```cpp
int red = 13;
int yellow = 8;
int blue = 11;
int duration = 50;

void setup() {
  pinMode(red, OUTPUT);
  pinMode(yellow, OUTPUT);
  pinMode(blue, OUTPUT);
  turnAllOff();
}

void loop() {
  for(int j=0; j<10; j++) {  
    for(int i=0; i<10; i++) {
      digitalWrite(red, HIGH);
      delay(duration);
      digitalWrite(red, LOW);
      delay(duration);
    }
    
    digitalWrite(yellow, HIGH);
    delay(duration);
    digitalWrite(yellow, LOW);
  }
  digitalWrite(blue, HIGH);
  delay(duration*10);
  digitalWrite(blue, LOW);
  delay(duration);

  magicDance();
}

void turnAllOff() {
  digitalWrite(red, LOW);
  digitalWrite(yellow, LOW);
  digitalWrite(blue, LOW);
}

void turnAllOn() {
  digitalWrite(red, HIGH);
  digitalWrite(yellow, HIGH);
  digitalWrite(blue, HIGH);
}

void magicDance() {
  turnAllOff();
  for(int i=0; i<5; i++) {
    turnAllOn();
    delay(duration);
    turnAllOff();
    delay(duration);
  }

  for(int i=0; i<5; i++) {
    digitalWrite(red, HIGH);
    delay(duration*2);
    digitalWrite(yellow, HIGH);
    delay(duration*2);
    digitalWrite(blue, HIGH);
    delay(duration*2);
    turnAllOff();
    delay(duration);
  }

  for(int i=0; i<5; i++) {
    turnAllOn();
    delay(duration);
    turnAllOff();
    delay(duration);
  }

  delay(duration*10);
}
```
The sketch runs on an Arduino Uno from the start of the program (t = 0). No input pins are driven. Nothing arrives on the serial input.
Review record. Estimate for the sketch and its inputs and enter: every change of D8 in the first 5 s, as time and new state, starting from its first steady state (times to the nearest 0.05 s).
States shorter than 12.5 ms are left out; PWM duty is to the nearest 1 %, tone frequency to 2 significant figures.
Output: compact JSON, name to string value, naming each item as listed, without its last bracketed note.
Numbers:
{"every change of D8 in the first 5 s, as time and new state, starting from its first steady state": "0 s low; 1 s high; 1.05 s low; 2.05 s high; 2.1 s low; 3.1 s high; 3.15 s low; 4.15 s high; 4.2 s low"}
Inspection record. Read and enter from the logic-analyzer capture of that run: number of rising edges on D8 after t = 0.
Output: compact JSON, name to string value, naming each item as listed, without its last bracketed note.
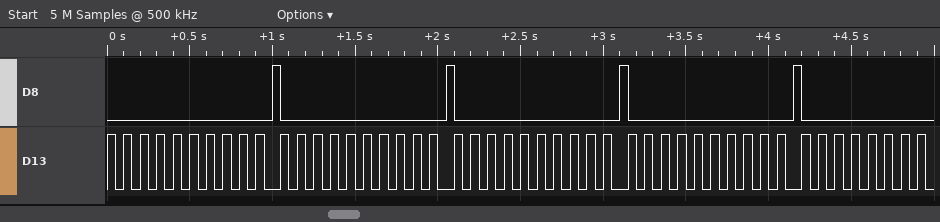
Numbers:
{"number of rising edges on D8 after t = 0": "4"}
